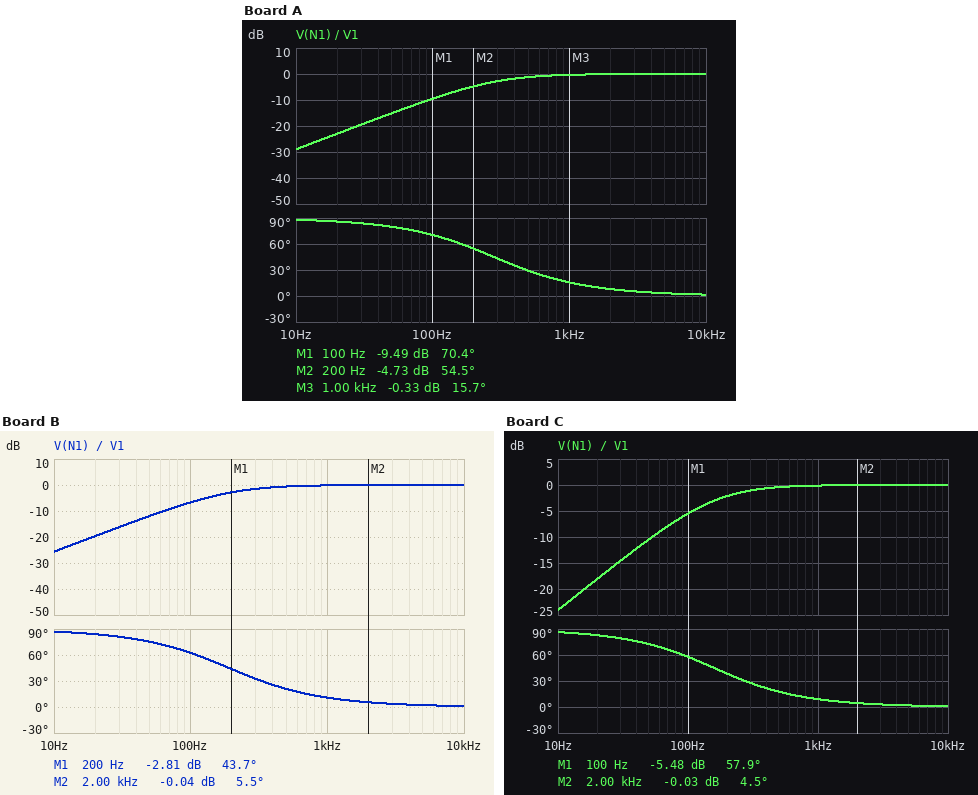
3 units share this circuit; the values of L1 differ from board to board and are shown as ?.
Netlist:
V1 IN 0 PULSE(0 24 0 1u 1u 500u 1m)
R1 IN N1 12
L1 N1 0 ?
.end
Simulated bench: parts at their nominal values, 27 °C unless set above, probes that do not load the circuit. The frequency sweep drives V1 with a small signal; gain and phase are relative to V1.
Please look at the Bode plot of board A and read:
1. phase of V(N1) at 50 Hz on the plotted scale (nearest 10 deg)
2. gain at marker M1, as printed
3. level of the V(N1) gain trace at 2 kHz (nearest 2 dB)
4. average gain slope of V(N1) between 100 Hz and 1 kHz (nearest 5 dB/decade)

80 deg
-9.49 dB
0 dB
10 dB/decade
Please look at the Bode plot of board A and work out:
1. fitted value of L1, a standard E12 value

6.8 mH
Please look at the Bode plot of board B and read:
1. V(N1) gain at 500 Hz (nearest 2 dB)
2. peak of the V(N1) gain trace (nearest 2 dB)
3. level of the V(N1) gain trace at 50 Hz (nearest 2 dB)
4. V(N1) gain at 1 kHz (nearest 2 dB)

0 dB
0 dB
-12 dB
0 dB
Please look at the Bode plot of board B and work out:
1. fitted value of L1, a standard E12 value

10 mH
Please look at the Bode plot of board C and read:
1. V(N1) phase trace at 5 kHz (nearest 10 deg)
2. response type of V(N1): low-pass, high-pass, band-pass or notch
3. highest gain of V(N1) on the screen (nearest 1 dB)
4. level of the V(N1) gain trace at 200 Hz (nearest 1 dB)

0 deg
high-pass
0 dB
-2 dB
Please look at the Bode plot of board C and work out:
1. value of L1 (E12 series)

12 mH
